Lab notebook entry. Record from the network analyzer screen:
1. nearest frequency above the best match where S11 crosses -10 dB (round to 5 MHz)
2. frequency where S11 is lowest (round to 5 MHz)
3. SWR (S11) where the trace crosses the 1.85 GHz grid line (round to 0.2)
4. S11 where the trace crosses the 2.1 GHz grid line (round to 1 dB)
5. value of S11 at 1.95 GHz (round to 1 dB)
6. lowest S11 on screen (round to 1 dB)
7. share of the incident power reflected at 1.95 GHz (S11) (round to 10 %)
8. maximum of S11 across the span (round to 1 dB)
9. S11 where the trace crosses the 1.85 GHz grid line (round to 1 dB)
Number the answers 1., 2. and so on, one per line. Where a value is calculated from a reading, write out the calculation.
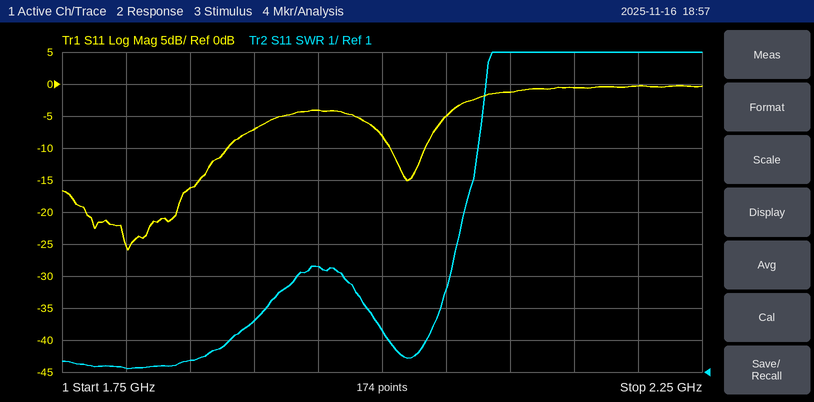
1. 1.880 GHz
2. 1.800 GHz
3. 1.4
4. -1 dB
5. -4 dB
6. -26 dB
7. 10^(-4/10) ≈ 40 %
8. 0 dB
9. -16 dB
